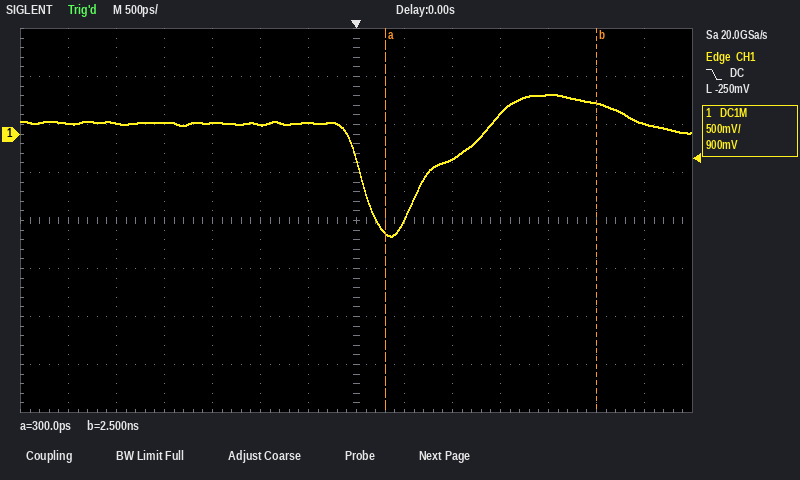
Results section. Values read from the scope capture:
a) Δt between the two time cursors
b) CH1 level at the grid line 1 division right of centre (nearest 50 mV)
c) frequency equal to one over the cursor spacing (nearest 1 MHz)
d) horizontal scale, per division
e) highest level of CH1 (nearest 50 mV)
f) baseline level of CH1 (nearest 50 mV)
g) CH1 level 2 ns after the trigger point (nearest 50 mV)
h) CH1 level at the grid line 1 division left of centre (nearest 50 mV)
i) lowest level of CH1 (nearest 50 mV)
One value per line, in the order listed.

2.20 ns
-900 mV
455 MHz
500 ps
400 mV
100 mV
400 mV
100 mV
-1.05 V
